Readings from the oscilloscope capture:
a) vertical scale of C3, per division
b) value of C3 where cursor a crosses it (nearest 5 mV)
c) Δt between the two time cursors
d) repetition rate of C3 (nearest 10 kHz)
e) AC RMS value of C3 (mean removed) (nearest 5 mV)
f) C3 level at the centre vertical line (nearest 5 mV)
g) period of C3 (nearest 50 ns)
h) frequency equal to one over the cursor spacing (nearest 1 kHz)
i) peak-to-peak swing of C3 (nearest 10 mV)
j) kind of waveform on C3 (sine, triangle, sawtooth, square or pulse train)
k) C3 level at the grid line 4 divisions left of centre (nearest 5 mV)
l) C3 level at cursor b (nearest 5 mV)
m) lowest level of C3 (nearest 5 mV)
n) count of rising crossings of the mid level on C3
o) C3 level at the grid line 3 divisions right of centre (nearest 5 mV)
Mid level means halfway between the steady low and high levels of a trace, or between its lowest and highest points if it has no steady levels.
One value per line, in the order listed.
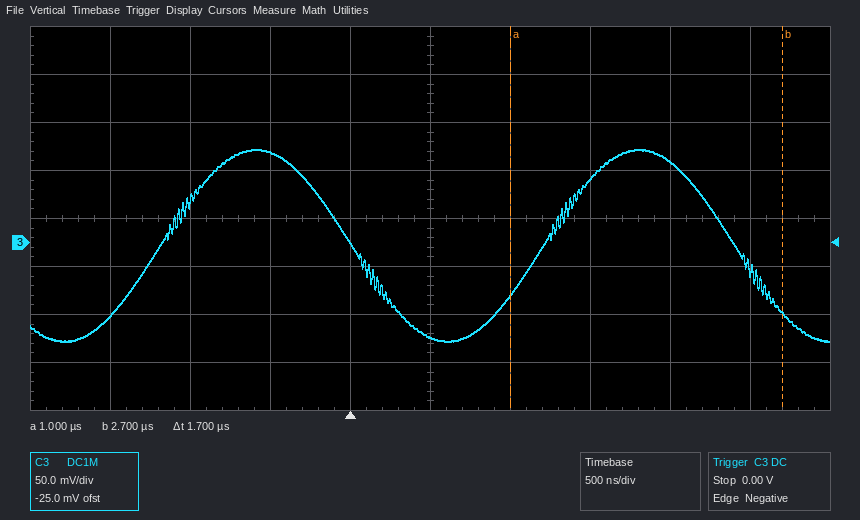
50 mV
-55 mV
1.7 µs
420 kHz
70 mV
-100 mV
2.40 µs
588 kHz
200 mV
sine
-75 mV
-75 mV
-105 mV
2
85 mV
